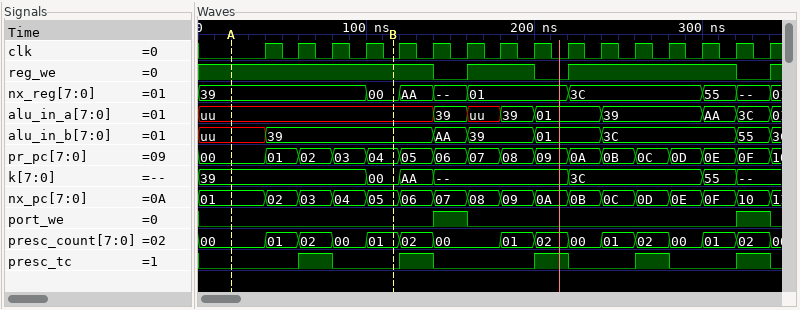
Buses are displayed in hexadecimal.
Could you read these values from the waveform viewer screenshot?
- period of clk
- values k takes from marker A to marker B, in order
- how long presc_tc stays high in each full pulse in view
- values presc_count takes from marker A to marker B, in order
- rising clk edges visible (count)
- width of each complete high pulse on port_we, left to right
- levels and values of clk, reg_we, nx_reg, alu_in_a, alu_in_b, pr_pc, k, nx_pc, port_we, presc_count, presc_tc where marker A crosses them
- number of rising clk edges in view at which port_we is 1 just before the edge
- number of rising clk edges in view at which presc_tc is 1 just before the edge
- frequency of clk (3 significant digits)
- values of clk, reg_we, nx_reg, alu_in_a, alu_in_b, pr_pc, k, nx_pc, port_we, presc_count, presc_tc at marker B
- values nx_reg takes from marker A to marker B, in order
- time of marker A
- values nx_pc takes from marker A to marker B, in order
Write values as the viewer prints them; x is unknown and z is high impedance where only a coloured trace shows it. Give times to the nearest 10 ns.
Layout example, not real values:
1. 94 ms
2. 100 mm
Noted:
1. 20 ns
2. 39, 00
3. 20 ns, 20 ns, 20 ns, 20 ns, 20 ns
4. 00, 01, 02, 00, 01
5. 16
6. 20 ns, 20 ns
7. clk=0, reg_we=1, nx_reg=39, alu_in_a=uu, alu_in_b=uu, pr_pc=00, k=39, nx_pc=01, port_we=0, presc_count=00, presc_tc=0
8. 2
9. 5
10. 50.0 MHz
11. clk=0, reg_we=1, nx_reg=00, alu_in_a=uu, alu_in_b=39, pr_pc=04, k=00, nx_pc=05, port_we=0, presc_count=01, presc_tc=0
12. 39, 00
13. 20 ns
14. 01, 02, 03, 04, 05
